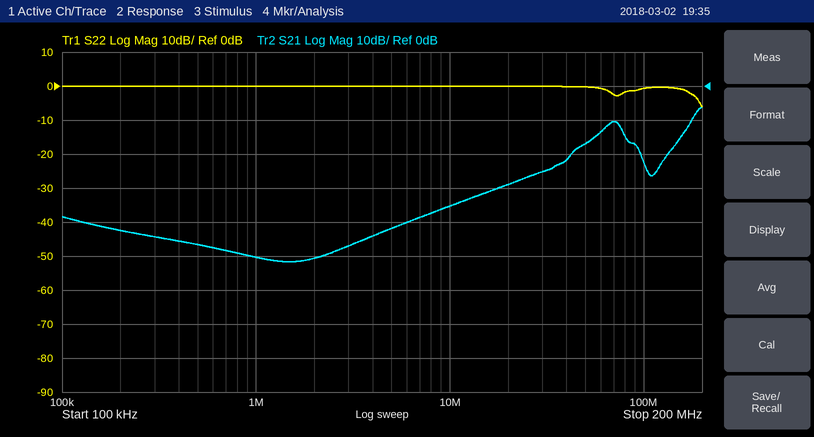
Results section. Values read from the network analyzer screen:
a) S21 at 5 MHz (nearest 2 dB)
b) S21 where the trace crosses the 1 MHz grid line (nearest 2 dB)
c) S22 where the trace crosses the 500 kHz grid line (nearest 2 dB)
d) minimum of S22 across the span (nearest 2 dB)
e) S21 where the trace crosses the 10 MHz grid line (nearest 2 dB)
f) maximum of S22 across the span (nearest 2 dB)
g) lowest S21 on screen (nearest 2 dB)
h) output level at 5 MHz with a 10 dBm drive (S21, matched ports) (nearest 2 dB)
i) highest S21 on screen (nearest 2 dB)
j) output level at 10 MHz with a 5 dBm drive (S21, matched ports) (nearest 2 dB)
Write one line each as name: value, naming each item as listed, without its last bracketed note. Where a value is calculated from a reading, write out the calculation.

S21 at 5 MHz: -42 dB
S21 where the trace crosses the 1 MHz grid line: -50 dB
S22 where the trace crosses the 500 kHz grid line: 0 dB
minimum of S22 across the span: -6 dB
S21 where the trace crosses the 10 MHz grid line: -36 dB
maximum of S22 across the span: 0 dB
lowest S21 on screen: -52 dB
output level at 5 MHz with a 10 dBm drive (S21, matched ports): 10 dBm + (-42 dB) = -32 dBm
highest S21 on screen: -6 dB
output level at 10 MHz with a 5 dBm drive (S21, matched ports): 5 dBm + (-36 dB) = -30 dBm
